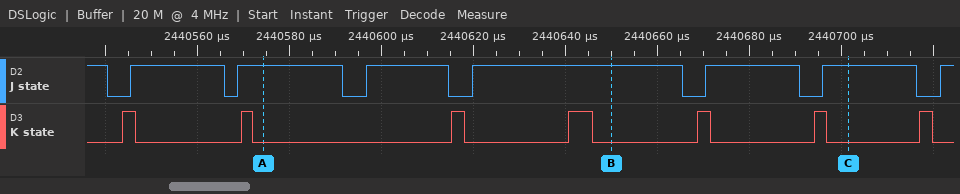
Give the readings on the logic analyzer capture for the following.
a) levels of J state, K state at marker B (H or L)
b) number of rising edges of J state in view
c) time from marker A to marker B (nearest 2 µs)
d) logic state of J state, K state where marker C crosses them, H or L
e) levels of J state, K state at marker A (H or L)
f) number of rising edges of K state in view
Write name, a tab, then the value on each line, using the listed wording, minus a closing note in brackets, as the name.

levels of J state, K state at marker B	J state=H, K state=L
number of rising edges of J state in view	7
time from marker A to marker B	76 µs
logic state of J state, K state where marker C crosses them, H or L	J state=H, K state=L
levels of J state, K state at marker A	J state=H, K state=L
number of rising edges of K state in view	7
